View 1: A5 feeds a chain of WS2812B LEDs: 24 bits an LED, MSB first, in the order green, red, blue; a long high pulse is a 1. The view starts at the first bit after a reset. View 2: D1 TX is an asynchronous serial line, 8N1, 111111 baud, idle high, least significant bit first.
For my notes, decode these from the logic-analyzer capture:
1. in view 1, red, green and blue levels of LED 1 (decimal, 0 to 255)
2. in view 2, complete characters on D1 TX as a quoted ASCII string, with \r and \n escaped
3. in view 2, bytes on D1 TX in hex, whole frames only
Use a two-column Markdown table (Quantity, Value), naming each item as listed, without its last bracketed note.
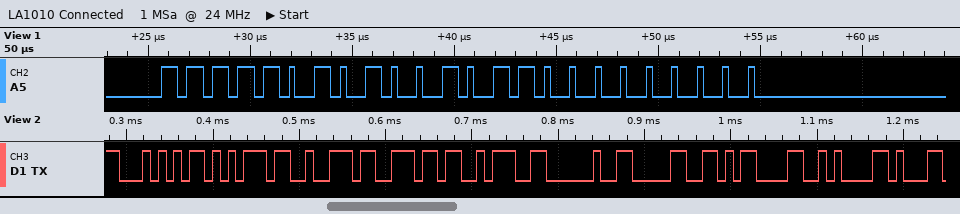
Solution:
| Quantity | Value |
|---|---|
| in view 1, red, green and blue levels of LED 1 | 150, 250, 0 |
| in view 2, complete characters on D1 TX as a quoted ASCII string, with \r and \n escaped | "Turn: 0\r\n" |
| in view 2, bytes on D1 TX in hex, whole frames only | 0x54 0x75 0x72 0x6E 0x3A 0x20 0x30 0x0D 0x0A |
